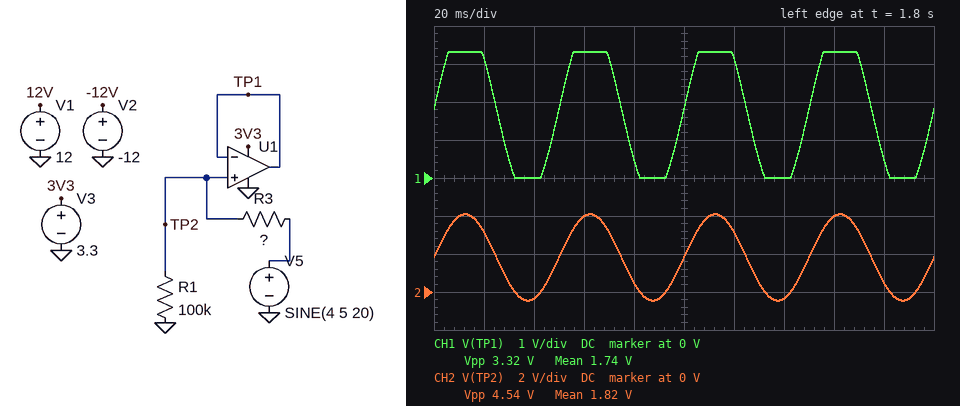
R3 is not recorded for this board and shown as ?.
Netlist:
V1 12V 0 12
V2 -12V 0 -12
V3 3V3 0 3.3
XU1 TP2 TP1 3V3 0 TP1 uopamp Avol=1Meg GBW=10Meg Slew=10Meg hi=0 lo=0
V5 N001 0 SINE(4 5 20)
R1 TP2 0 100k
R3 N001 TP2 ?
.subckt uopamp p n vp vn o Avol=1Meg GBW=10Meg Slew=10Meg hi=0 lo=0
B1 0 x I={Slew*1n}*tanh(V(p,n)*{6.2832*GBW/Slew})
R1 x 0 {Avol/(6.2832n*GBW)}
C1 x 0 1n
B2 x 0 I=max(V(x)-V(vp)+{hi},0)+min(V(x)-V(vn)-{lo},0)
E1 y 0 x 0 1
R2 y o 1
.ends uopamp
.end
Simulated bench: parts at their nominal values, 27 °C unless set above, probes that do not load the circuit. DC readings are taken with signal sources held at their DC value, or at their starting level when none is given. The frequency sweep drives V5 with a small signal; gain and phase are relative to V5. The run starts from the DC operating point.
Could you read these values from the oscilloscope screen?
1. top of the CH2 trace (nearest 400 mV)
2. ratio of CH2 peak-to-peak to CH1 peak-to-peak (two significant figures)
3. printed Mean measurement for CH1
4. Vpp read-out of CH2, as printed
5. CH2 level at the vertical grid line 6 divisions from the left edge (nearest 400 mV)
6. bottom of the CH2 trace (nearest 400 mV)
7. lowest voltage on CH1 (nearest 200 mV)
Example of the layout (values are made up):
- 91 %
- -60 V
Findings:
- 4.0 V
- 1.4
- 1.74 V
- 4.54 V
- 3.2 V
- -400 mV
- 0 V
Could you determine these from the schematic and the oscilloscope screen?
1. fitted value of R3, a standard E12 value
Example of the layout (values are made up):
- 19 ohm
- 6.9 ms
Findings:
- 120 kΩ
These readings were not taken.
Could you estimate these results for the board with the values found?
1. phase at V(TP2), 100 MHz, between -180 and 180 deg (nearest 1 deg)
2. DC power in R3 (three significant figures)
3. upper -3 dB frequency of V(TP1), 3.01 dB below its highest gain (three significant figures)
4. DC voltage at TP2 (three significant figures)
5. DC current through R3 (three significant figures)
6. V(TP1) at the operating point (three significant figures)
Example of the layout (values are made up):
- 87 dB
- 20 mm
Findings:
- 0 deg
- 39.7 µW
- 10.0 MHz
- 1.82 V
- 18.2 µA
- 1.82 V
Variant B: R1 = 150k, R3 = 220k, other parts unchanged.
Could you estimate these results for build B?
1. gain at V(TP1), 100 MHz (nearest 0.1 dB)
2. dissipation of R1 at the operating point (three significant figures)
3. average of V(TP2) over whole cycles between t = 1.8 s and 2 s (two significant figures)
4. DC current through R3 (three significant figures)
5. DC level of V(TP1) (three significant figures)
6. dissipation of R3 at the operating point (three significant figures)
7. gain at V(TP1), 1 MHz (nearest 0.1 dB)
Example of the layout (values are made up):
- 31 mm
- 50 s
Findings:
- -27.9 dB
- 17.5 µW
- 1.6 V
- 10.8 µA
- 1.62 V
- 25.7 µW
- -7.9 dB
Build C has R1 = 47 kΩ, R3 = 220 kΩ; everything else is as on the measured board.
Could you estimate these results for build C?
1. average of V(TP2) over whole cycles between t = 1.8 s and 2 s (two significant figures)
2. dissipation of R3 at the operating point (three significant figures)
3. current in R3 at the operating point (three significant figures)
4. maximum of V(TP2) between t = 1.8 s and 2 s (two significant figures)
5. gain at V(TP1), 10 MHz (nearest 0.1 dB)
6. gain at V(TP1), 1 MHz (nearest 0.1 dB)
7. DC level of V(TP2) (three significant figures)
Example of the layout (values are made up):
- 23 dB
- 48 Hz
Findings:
- 700 mV
- 49.4 µW
- 15.0 µA
- 1.6 V
- -18.1 dB
- -15.1 dB
- 704 mV
